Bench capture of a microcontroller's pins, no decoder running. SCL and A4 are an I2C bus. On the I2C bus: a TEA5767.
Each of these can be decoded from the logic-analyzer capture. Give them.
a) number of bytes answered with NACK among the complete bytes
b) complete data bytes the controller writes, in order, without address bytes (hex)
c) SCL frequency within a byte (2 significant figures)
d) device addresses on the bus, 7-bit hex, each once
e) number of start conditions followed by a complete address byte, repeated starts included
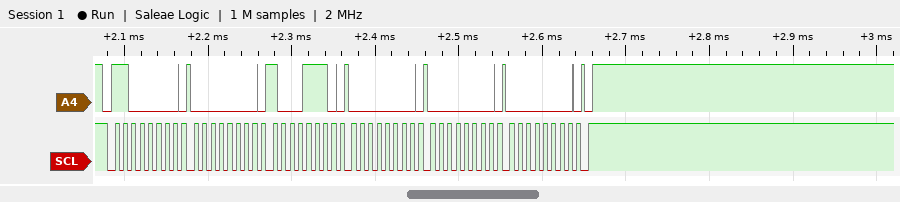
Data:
0
00 8E 00 00 00
100 kHz
0x60
1
